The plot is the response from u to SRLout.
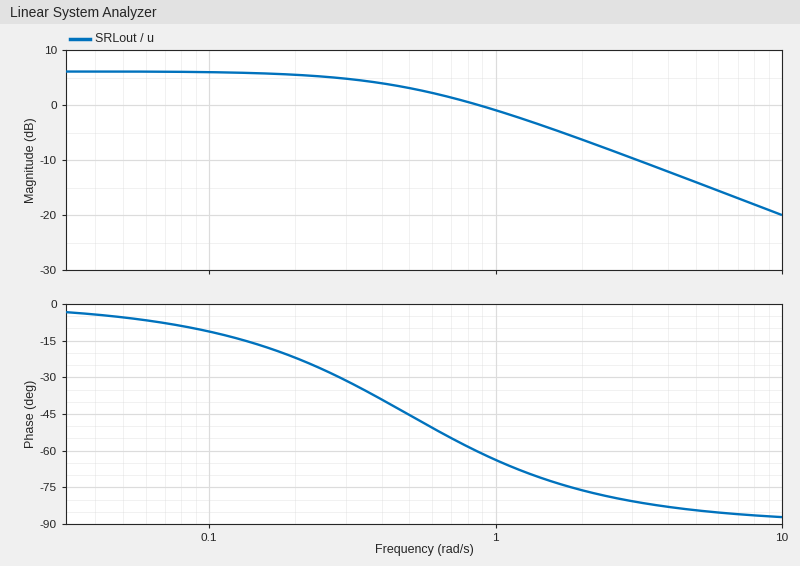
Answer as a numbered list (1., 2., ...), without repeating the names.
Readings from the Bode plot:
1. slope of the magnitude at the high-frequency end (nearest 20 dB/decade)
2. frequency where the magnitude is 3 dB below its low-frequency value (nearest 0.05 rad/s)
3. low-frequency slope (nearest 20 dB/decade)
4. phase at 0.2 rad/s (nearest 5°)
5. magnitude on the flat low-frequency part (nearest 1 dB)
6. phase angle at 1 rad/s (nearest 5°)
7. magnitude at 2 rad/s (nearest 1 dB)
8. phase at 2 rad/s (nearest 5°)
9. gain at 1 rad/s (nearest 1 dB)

1. -20 dB/decade
2. 0.50 rad/s
3. 0 dB/decade
4. -20°
5. 6 dB
6. -65°
7. -6 dB
8. -75°
9. -1 dB
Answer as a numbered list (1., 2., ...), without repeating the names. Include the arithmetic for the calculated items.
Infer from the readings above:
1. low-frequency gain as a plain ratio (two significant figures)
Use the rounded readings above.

1. 10^(6 / 20) = 2.0
